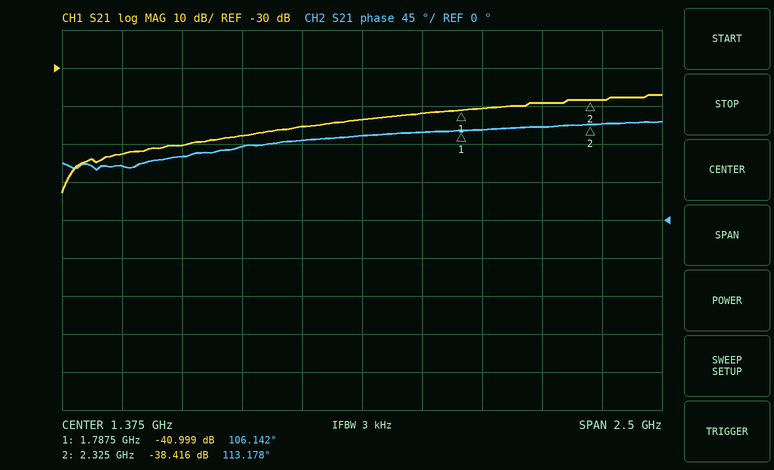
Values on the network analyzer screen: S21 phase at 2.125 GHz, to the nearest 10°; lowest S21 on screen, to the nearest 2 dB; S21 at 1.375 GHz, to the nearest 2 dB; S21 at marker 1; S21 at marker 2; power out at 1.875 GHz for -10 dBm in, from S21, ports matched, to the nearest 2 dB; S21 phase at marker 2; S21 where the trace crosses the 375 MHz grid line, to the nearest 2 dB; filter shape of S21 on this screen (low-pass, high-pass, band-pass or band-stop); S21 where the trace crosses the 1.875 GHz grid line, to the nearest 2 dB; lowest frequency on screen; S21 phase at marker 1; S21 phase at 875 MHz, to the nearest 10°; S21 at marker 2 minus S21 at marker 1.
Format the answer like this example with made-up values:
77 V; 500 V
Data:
110°; -62 dB; -44 dB; -40.999 dB; -38.416 dB; -50 dBm; 113.178°; -52 dB; high-pass; -40 dB; 125 MHz; 106.142°; 90°; 2.583 dB
